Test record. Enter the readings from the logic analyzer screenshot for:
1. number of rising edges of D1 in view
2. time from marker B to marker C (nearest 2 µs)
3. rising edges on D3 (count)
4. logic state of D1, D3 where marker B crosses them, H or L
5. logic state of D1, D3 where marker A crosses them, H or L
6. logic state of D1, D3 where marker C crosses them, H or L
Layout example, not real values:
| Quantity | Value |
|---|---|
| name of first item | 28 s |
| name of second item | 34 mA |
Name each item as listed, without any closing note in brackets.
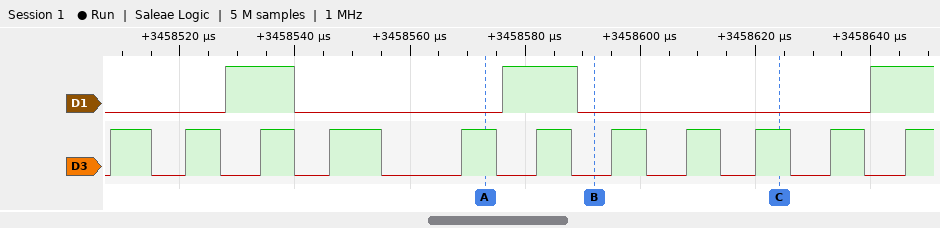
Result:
| Quantity | Value |
|---|---|
| number of rising edges of D1 in view | 3 |
| time from marker B to marker C | 32 µs |
| rising edges on D3 | 11 |
| logic state of D1, D3 where marker B crosses them, H or L | D1=L, D3=L |
| logic state of D1, D3 where marker A crosses them, H or L | D1=L, D3=H |
| logic state of D1, D3 where marker C crosses them, H or L | D1=L, D3=H |
